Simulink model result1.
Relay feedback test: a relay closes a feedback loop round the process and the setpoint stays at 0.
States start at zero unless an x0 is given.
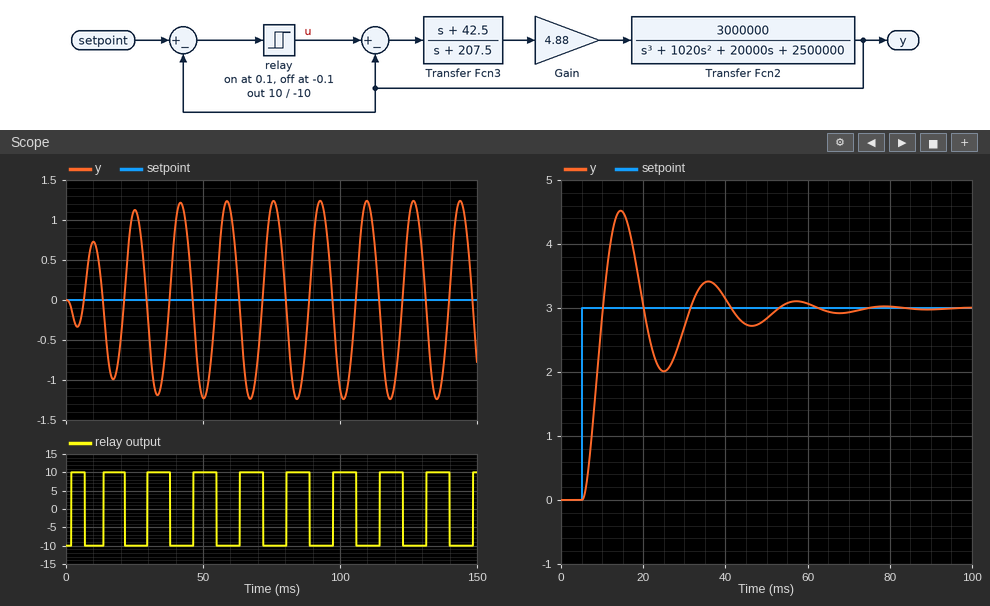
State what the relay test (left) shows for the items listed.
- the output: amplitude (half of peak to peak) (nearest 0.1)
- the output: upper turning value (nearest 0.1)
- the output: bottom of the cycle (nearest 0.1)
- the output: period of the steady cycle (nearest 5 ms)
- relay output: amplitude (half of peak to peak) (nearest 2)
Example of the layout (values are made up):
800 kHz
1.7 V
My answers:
1.2
1.2
-1.2
15 ms
10
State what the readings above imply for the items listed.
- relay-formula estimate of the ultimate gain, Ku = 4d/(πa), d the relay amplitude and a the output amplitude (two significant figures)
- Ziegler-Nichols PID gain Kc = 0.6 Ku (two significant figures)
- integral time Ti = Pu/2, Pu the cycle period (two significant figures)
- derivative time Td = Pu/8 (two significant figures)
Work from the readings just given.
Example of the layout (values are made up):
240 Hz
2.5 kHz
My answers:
11
6.6
7.5 ms
1.9 ms
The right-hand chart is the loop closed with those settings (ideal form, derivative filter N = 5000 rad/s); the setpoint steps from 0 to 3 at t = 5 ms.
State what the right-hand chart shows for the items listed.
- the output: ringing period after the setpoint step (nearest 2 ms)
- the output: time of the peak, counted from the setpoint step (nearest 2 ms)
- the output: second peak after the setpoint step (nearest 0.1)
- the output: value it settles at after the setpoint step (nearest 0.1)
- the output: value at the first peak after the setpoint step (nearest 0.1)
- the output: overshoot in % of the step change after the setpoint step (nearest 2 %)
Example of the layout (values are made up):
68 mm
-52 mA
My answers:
22 ms
10 ms
3.4
3.0
4.5
50 %
